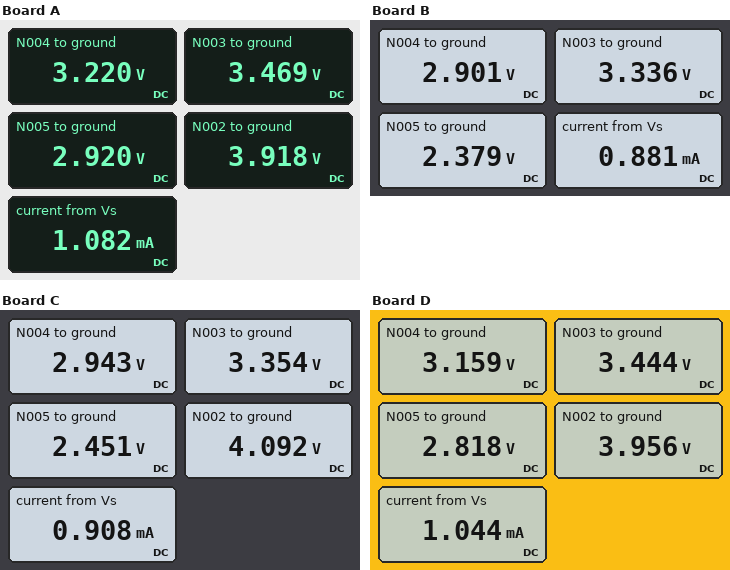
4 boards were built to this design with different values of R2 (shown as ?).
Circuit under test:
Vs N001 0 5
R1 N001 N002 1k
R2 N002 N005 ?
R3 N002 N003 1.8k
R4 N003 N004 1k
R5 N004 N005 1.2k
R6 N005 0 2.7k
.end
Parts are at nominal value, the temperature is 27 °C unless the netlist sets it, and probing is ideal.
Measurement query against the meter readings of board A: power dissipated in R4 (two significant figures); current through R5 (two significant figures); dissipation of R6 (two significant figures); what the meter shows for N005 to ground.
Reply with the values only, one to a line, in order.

62 µW
250 µA
3.2 mW
2.920 V
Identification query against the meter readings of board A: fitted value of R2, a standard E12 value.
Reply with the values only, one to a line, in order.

1.2 kΩ
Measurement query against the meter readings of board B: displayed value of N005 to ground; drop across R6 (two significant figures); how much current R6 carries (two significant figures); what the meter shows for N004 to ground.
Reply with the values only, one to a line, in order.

2.379 V
2.4 V
880 µA
2.901 V
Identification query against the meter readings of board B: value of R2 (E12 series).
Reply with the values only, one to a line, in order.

3.9 kΩ
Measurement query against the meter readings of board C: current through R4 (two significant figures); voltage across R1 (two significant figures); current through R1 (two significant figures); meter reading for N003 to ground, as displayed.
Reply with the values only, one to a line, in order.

410 µA
910 mV
910 µA
3.354 V
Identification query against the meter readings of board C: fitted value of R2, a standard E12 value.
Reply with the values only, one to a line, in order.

3.3 kΩ
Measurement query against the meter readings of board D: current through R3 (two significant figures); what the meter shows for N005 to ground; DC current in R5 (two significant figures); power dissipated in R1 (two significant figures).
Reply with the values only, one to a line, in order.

280 µA
2.818 V
280 µA
1.1 mW
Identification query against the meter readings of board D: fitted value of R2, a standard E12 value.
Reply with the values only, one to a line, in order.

1.5 kΩ
